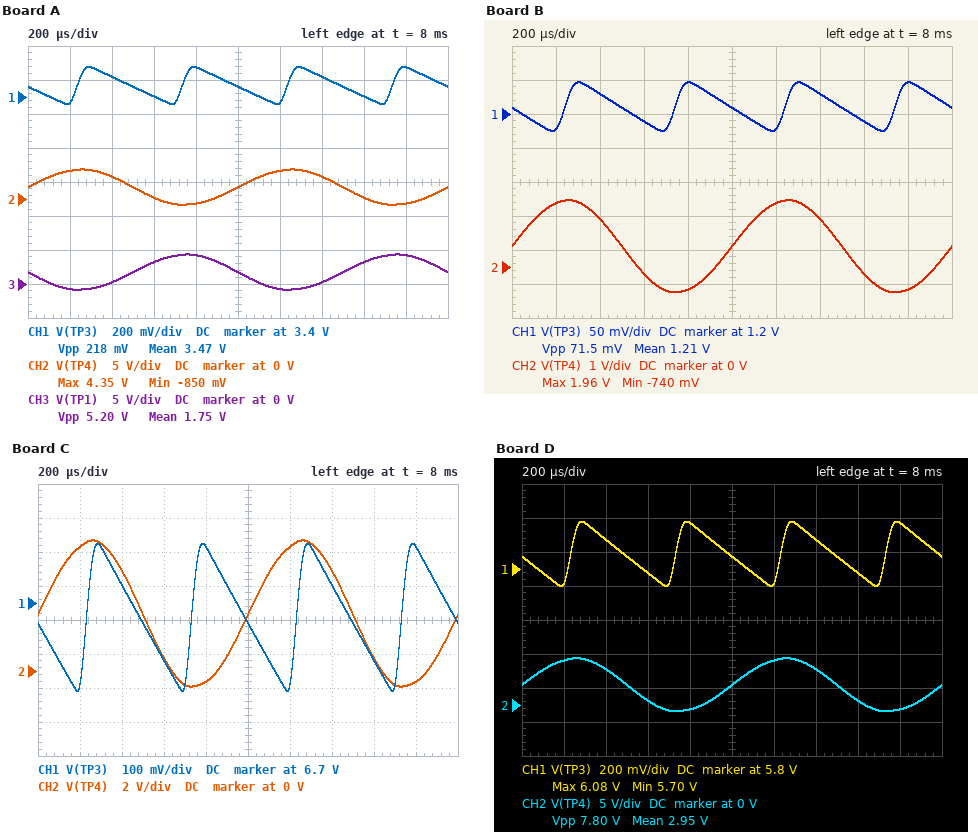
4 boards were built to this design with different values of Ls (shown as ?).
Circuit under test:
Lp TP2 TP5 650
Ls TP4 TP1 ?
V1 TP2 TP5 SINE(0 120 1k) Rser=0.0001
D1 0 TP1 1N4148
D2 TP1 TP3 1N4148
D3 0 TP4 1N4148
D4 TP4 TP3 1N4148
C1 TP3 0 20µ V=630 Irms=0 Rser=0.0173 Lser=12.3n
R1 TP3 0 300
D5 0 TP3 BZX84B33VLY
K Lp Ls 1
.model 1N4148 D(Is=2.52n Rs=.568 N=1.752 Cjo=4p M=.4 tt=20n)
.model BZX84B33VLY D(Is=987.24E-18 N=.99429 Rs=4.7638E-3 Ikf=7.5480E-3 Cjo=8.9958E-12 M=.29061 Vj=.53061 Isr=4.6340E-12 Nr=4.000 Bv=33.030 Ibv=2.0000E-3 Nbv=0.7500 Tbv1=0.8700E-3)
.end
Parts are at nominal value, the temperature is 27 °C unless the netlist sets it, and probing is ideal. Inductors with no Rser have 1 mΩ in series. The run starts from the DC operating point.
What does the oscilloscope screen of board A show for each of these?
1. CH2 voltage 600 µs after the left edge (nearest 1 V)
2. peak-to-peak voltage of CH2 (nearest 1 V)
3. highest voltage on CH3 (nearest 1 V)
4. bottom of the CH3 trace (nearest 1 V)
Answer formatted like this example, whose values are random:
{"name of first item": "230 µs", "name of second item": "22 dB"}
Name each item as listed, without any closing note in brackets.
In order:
{"CH2 voltage 600 µs after the left edge": "0 V", "peak-to-peak voltage of CH2": "5 V", "highest voltage on CH3": "4 V", "bottom of the CH3 trace": "-1 V"}
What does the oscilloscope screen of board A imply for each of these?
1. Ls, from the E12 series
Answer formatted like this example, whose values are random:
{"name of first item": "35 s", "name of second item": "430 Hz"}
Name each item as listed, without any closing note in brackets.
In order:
{"Ls, from the E12 series": "1.2 H"}
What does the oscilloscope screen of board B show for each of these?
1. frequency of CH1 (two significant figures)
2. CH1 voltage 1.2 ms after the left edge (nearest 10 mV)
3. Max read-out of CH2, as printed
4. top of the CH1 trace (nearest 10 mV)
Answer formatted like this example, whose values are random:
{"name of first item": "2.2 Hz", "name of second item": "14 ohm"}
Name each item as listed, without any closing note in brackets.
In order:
{"frequency of CH1": "2.0 kHz", "CH1 voltage 1.2 ms after the left edge": "1.18 V", "Max read-out of CH2, as printed": "1.96 V", "top of the CH1 trace": "1.25 V"}
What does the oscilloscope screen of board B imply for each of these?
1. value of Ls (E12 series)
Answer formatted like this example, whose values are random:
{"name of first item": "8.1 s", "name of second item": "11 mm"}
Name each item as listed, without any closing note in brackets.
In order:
{"value of Ls": "330 mH"}
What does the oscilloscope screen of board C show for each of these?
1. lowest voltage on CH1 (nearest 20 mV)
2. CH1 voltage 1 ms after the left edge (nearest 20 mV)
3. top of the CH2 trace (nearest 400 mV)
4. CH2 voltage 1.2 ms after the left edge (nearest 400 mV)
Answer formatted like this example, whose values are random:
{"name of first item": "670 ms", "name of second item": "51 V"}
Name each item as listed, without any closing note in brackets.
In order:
{"lowest voltage on CH1": "6.44 V", "CH1 voltage 1 ms after the left edge": "6.64 V", "top of the CH2 trace": "7.6 V", "CH2 voltage 1.2 ms after the left edge": "7.2 V"}
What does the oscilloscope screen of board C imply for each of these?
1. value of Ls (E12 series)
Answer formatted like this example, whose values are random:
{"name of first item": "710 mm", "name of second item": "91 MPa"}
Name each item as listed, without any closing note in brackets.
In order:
{"value of Ls": "3.3 H"}
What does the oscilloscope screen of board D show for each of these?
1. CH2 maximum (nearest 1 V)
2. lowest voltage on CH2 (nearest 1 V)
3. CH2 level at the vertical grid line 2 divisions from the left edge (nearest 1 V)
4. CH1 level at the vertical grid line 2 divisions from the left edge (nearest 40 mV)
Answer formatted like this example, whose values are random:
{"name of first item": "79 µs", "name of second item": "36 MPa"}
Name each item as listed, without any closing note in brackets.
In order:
{"CH2 maximum": "7 V", "lowest voltage on CH2": "-1 V", "CH2 level at the vertical grid line 2 divisions from the left edge": "5 V", "CH1 level at the vertical grid line 2 divisions from the left edge": "5.96 V"}
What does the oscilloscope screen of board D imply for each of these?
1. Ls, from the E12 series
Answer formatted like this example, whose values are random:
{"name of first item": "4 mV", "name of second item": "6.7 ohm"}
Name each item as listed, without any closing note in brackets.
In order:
{"Ls, from the E12 series": "2.7 H"}
